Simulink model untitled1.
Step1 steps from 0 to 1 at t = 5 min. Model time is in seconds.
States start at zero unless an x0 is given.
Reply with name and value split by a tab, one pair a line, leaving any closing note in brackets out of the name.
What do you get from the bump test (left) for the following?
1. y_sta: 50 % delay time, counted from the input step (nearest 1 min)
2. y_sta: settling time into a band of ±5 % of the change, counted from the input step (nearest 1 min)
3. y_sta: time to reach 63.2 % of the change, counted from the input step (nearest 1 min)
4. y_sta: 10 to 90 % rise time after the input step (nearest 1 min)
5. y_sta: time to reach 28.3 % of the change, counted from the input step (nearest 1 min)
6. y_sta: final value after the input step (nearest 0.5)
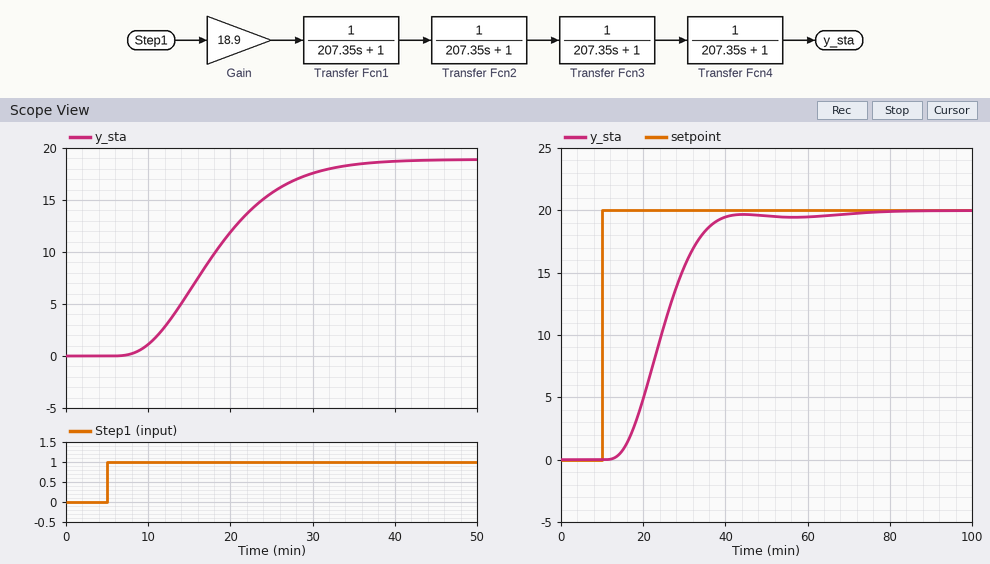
y_sta: 50 % delay time, counted from the input step	13 min
y_sta: settling time into a band of ±5 % of the change, counted from the input step	27 min
y_sta: time to reach 63.2 % of the change, counted from the input step	15 min
y_sta: 10 to 90 % rise time after the input step	17 min
y_sta: time to reach 28.3 % of the change, counted from the input step	9 min
y_sta: final value after the input step	19.0
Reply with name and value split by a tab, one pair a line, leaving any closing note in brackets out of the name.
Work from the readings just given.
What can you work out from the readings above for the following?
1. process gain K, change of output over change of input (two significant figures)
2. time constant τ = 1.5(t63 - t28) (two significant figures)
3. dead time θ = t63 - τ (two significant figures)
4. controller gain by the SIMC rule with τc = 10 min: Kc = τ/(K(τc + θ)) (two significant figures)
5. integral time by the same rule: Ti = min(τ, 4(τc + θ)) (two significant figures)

process gain K, change of output over change of input	19
time constant τ = 1.5(t63 - t28)	9.0 min
dead time θ = t63 - τ	6.0 min
controller gain by the SIMC rule with τc = 10 min: Kc = τ/(K(τc + θ))	0.030
integral time by the same rule: Ti = min(τ, 4(τc + θ))	9.0 min
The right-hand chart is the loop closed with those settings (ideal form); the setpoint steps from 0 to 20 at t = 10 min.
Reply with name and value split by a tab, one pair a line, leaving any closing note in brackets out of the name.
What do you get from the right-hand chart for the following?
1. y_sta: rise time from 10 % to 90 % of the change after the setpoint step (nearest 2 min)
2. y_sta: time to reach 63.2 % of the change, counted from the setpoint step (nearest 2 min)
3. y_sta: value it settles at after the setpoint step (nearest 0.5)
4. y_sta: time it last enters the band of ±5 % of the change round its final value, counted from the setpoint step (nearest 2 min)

y_sta: rise time from 10 % to 90 % of the change after the setpoint step	18 min
y_sta: time to reach 63.2 % of the change, counted from the setpoint step	16 min
y_sta: value it settles at after the setpoint step	20.0
y_sta: time it last enters the band of ±5 % of the change round its final value, counted from the setpoint step	28 min
